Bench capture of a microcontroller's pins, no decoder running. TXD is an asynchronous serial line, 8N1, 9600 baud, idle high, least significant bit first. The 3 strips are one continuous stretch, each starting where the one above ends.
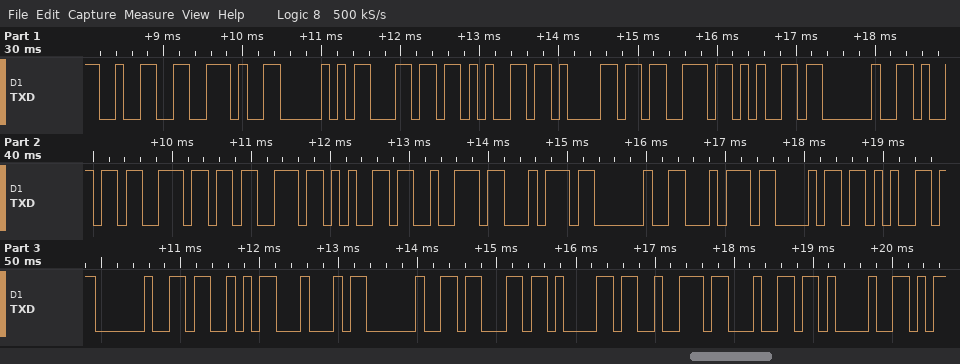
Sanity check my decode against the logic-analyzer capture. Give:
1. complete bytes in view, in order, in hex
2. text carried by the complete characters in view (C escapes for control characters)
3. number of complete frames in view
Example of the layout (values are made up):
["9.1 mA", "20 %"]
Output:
["0x32 0x2E 0x50 0x6C 0x65 0x61 0x73 0x65 0x20 0x69 0x6E 0x73 0x65 0x72 0x74 0x20 0x74 0x68 0x65 0x20 0x53 0x44 0x20 0x63 0x61 0x72 0x64 0x21", "\"2.Please insert the SD card!\"", "28"]
